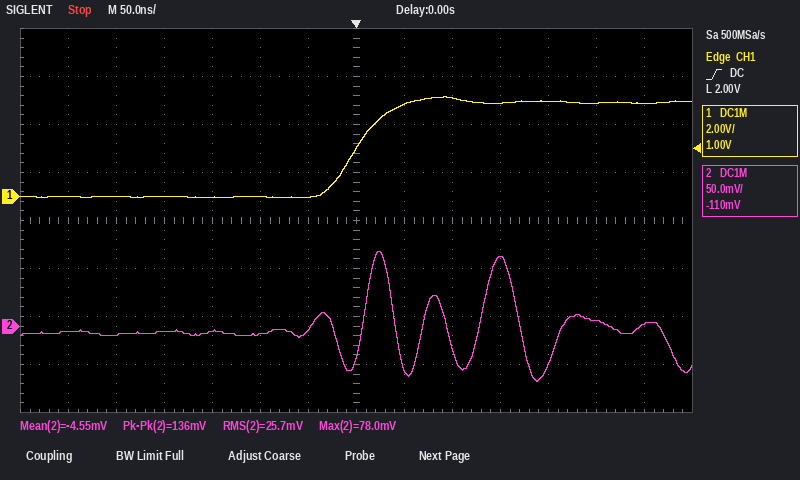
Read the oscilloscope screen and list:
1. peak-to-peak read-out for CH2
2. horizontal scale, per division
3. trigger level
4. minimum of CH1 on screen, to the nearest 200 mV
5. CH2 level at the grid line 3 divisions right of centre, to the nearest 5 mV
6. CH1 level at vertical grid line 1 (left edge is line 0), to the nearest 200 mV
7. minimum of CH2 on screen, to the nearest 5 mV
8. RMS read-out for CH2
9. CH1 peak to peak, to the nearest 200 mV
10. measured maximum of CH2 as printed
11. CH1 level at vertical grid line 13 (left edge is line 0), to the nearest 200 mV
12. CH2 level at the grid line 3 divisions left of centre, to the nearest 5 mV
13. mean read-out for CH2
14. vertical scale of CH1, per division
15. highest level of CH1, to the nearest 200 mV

136 mV
50 ns
2.00 V
0.0 V
70 mV
0.0 V
-60 mV
25.7 mV
4.2 V
78.0 mV
3.8 V
-5 mV
-4.55 mV
2 V
4.2 V
